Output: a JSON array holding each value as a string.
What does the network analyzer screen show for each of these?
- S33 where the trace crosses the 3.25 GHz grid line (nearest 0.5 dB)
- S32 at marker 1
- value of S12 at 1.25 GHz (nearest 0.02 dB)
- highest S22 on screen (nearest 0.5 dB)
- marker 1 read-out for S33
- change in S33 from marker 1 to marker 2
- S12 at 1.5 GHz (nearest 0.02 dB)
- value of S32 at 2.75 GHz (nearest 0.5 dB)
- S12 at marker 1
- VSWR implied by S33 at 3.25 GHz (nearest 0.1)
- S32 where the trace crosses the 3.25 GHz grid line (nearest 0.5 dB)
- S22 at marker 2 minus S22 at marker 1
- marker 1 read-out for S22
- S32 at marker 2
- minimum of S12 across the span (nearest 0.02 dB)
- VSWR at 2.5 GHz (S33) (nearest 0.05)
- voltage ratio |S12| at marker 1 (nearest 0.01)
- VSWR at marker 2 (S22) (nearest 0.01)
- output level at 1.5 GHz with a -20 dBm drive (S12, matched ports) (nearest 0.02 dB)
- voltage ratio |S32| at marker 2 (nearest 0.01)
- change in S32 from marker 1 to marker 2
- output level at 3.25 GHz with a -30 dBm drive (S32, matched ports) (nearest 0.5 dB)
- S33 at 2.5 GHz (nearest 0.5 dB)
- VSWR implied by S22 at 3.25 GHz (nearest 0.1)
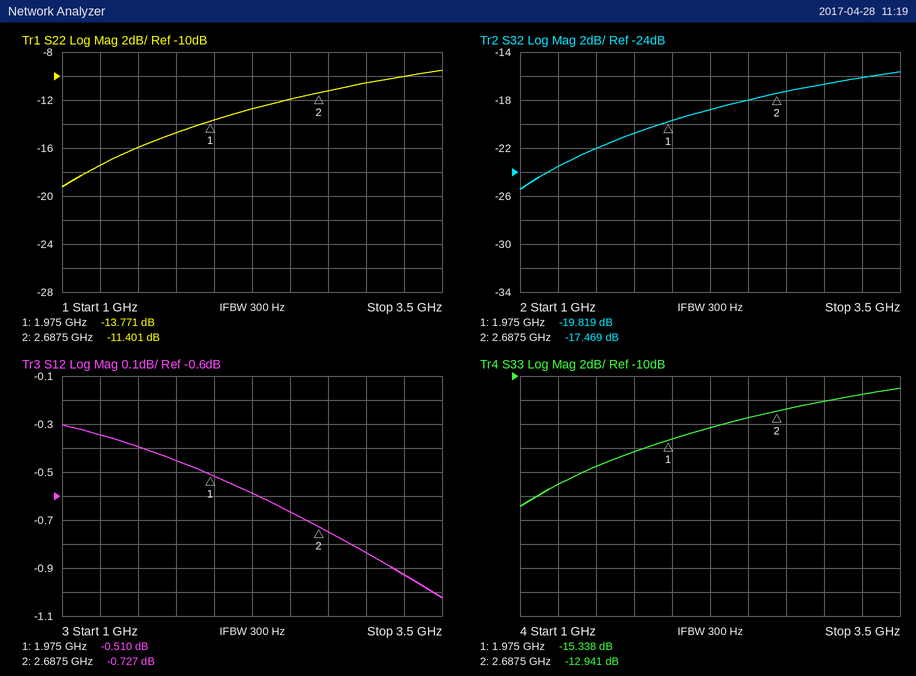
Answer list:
["-11.5 dB", "-19.819 dB", "-0.34 dB", "-9.5 dB", "-15.338 dB", "2.397 dB", "-0.40 dB", "-17.5 dB", "-0.510 dB", "1.7", "-16.0 dB", "2.370 dB", "-13.771 dB", "-17.469 dB", "-1.02 dB", "1.55", "0.94", "1.74", "-20.40 dBm", "0.13", "2.350 dB", "-46.0 dBm", "-13.5 dB", "1.9"]
